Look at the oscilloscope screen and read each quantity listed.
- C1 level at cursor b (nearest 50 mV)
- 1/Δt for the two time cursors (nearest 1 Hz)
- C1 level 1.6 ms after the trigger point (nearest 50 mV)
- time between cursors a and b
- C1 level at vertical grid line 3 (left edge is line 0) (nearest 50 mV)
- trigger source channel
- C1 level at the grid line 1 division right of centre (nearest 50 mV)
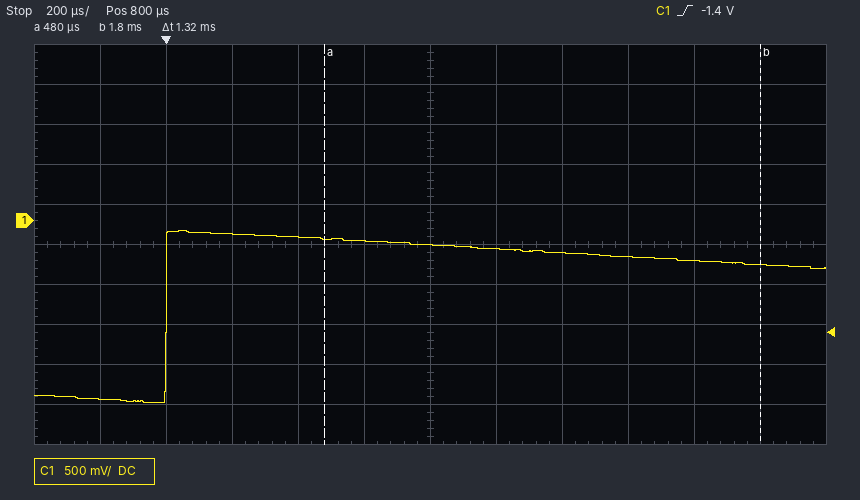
-550 mV
758 Hz
-500 mV
1.32 ms
-150 mV
C1
-350 mV
